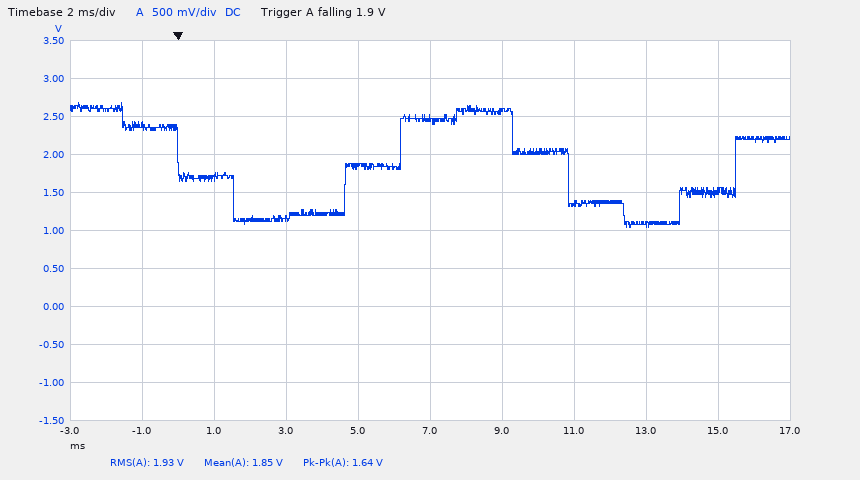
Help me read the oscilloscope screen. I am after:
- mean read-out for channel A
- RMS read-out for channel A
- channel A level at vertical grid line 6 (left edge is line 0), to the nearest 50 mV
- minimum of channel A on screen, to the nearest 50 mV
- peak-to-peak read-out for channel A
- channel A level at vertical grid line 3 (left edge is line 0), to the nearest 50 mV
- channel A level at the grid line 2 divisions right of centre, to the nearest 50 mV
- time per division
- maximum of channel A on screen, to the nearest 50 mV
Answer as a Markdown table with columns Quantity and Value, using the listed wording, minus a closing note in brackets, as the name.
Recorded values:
| Quantity | Value |
|---|---|
| mean read-out for channel A | 1.85 V |
| RMS read-out for channel A | 1.93 V |
| channel A level at vertical grid line 6 (left edge is line 0), to the nearest 50 mV | 2.55 V |
| minimum of channel A on screen, to the nearest 50 mV | 1.05 V |
| peak-to-peak read-out for channel A | 1.64 V |
| channel A level at vertical grid line 3 (left edge is line 0), to the nearest 50 mV | 1.15 V |
| channel A level at the grid line 2 divisions right of centre, to the nearest 50 mV | 1.35 V |
| time per division | 2 ms |
| maximum of channel A on screen, to the nearest 50 mV | 2.70 V |
